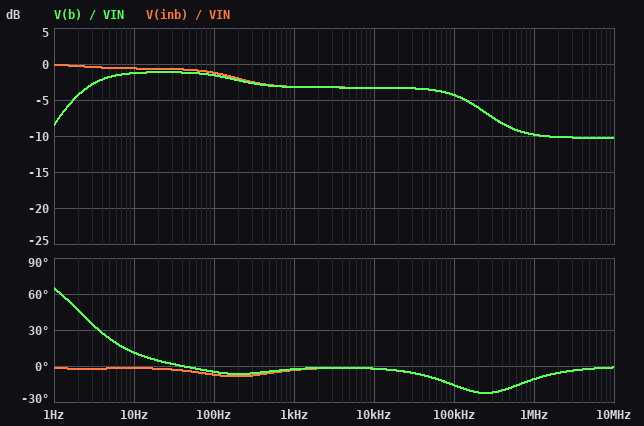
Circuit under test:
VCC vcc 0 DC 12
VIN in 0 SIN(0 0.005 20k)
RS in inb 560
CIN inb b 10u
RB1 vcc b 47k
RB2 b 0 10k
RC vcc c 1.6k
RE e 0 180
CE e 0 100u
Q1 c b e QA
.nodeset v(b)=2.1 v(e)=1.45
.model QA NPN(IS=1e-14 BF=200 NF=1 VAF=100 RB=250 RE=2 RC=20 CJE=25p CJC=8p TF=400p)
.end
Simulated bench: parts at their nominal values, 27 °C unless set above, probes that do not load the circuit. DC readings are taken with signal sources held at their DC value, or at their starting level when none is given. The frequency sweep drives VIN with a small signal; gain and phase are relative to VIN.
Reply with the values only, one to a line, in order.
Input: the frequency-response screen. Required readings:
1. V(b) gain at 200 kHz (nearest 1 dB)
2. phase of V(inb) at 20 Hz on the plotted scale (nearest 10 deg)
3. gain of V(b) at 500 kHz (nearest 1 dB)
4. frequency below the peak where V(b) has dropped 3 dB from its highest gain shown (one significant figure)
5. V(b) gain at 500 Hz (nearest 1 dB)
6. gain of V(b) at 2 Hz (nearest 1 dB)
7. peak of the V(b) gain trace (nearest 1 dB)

-6 dB
0 deg
-9 dB
2 Hz
-3 dB
-4 dB
-1 dB
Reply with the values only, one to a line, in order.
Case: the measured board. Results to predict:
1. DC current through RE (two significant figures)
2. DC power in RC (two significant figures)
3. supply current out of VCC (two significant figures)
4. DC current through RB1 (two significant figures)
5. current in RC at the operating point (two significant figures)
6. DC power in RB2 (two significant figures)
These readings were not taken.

6.3 mA
62 mW
6.4 mA
220 µA
6.2 mA
340 µW
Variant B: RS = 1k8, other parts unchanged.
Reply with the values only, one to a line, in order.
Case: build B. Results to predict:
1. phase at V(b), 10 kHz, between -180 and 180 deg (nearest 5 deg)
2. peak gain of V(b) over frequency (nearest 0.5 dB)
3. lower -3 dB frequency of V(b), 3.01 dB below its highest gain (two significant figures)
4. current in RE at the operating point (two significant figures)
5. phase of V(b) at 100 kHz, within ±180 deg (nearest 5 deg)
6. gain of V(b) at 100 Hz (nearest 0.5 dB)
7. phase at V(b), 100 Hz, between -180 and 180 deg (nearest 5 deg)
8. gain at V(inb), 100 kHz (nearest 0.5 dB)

-5 deg
-2.5 dB
1.8 Hz
6.3 mA
-25 deg
-4.0 dB
-15 deg
-10.0 dB
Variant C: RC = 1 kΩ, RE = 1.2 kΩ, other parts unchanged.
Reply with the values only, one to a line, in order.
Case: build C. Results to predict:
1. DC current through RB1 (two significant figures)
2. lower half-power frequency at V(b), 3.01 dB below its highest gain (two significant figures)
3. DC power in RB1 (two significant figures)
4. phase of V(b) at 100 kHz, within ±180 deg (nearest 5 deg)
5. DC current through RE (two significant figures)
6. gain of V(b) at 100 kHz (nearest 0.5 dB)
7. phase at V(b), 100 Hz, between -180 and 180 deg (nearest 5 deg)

210 µA
1.8 Hz
2.1 mW
-5 deg
1.2 mA
-1.5 dB
0 deg
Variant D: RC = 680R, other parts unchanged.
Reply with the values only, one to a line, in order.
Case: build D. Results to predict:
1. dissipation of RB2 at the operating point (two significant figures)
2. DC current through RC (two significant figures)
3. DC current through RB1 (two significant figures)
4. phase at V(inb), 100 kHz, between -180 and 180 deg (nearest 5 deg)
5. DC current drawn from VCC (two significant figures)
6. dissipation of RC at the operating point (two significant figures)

350 µW
6.3 mA
220 µA
-5 deg
6.5 mA
27 mW
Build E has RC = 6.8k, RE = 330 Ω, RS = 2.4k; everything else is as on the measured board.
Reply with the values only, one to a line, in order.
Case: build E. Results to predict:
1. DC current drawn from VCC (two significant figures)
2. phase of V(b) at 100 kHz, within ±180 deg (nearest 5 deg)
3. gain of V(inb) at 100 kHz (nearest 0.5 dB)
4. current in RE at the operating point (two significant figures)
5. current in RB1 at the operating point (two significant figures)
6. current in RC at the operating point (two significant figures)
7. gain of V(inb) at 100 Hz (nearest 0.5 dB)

1.9 mA
0 deg
-20.0 dB
1.8 mA
230 µA
1.7 mA
-18.5 dB
